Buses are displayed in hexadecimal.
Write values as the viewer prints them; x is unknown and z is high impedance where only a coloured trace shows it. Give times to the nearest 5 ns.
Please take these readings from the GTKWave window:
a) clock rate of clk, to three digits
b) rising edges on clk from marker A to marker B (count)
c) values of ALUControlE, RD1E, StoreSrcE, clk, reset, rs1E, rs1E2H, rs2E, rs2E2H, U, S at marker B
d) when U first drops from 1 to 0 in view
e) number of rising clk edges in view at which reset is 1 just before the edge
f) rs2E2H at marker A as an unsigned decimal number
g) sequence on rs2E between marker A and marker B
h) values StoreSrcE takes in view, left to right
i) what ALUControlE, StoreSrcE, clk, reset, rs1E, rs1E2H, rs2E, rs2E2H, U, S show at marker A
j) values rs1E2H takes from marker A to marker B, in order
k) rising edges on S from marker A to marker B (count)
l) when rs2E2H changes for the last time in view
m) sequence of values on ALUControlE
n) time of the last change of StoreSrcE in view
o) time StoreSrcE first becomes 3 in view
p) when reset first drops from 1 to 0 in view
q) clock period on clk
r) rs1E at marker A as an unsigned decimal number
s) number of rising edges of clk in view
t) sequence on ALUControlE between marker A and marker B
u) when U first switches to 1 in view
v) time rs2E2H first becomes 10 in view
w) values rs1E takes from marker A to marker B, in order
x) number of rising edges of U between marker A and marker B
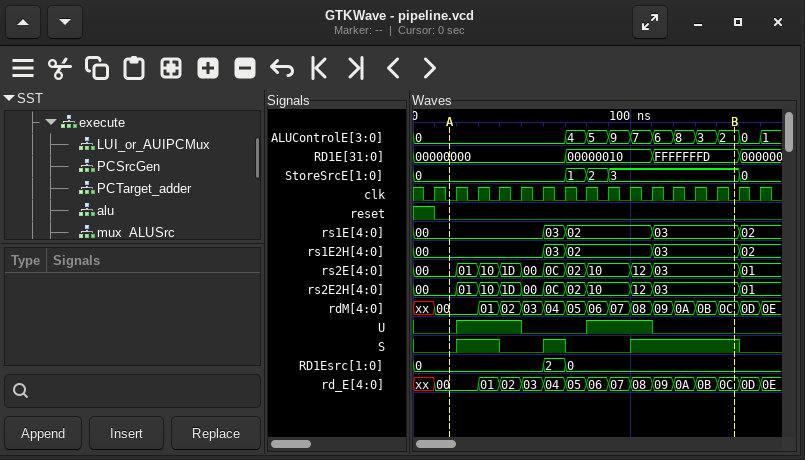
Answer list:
100 MHz
13
ALUControlE=2, RD1E=FFFFFFFD, StoreSrcE=3, clk=0, reset=0, rs1E=03, rs1E2H=03, rs2E=03, rs2E2H=03, U=0, S=1
50 ns
1
0
00, 01, 10, 1D, 00, 0C, 02, 10, 12, 03
0, 1, 2, 3, 0
ALUControlE=0, StoreSrcE=0, clk=0, reset=0, rs1E=00, rs1E2H=00, rs2E=00, rs2E2H=00, U=0, S=0
00, 03, 02, 03
3
150 ns
0, 4, 5, 9, 7, 6, 8, 3, 2, 0, 1
150 ns
90 ns
10 ns
10 ns
0
16
0, 4, 5, 9, 7, 6, 8, 3, 2
20 ns
30 ns
00, 03, 02, 03
2
